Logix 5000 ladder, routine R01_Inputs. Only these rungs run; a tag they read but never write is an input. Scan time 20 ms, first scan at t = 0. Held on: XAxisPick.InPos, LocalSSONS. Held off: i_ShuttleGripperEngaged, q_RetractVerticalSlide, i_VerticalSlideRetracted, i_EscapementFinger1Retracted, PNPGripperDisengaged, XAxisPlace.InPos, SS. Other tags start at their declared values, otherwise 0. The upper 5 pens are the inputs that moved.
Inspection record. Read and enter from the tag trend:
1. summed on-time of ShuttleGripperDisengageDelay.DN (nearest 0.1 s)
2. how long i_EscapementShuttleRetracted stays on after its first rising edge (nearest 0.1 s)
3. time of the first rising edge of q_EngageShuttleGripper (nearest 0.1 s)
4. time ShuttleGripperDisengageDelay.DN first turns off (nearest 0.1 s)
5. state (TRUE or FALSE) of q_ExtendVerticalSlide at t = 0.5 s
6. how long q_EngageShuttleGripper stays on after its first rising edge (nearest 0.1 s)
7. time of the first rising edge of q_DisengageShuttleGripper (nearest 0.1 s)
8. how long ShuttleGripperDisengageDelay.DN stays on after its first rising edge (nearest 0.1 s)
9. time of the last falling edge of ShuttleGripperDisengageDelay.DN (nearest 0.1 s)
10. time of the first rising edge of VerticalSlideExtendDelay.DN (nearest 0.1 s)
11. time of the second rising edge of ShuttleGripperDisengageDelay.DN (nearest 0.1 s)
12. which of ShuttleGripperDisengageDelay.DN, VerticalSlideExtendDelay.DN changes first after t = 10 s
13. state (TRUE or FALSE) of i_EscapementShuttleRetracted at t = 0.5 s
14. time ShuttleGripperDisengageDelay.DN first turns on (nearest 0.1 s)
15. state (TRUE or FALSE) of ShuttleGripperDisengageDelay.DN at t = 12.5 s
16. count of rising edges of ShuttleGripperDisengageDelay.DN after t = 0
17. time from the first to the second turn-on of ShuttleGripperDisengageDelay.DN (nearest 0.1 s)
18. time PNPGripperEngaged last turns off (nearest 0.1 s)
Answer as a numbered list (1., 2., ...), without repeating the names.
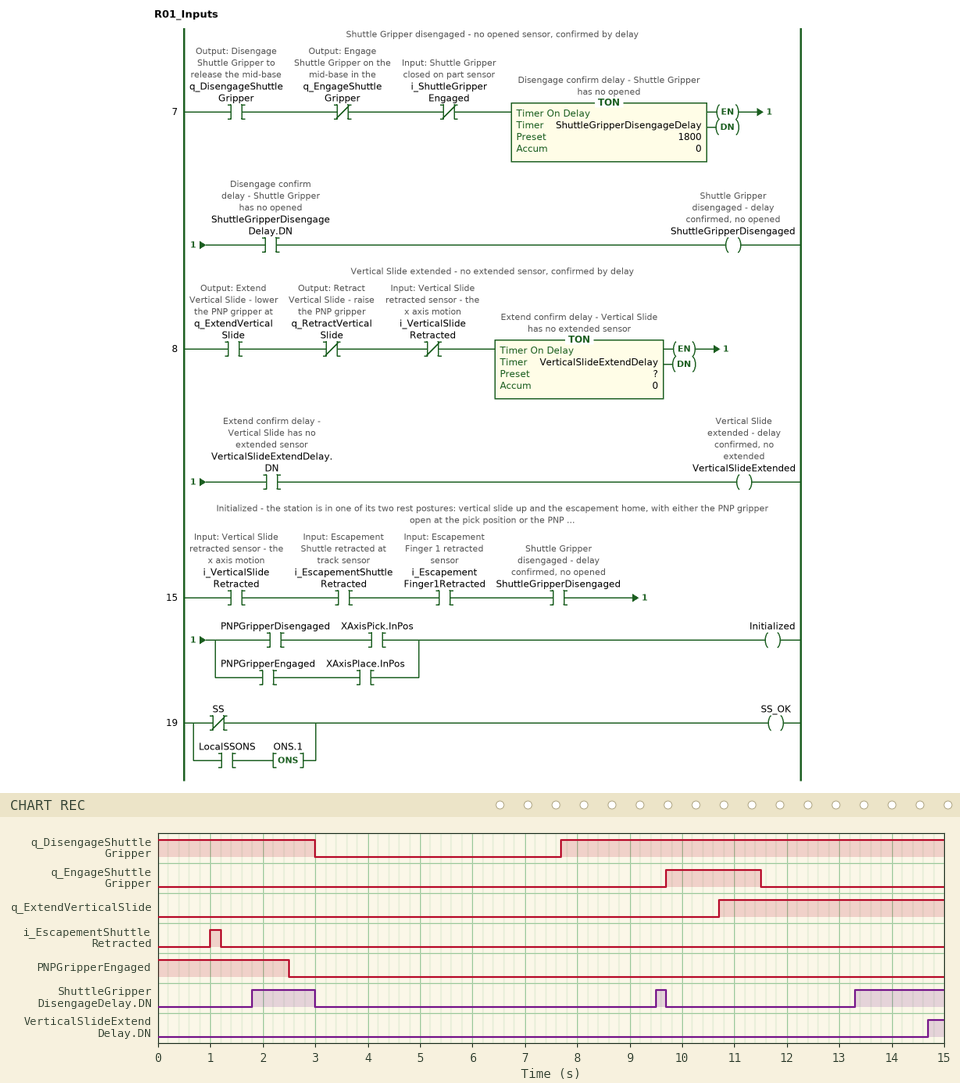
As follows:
1. 3.1 s
2. 0.2 s
3. 9.7 s
4. 3.0 s
5. FALSE
6. 1.8 s
7. 7.7 s
8. 1.2 s
9. 9.7 s
10. 14.7 s
11. 9.5 s
12. ShuttleGripperDisengageDelay.DN
13. FALSE
14. 1.8 s
15. FALSE
16. 3
17. 7.7 s
18. 2.5 s
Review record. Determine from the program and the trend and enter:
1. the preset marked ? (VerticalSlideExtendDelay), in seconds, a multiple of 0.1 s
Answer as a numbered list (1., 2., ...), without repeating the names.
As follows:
1. 4.0 s
